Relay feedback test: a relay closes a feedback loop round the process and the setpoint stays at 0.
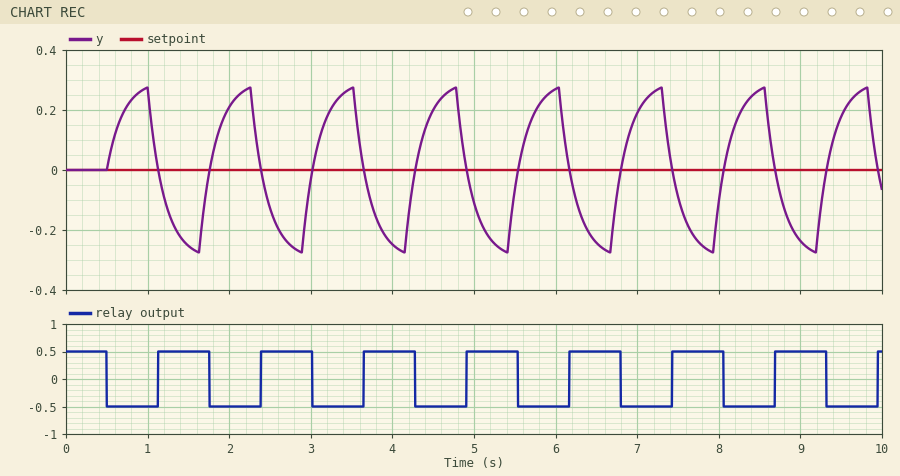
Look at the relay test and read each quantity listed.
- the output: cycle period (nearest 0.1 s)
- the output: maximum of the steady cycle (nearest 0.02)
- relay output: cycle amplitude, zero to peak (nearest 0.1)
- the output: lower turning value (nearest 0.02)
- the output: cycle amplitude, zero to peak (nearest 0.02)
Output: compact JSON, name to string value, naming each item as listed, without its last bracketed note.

{"the output: cycle period": "1.3 s", "the output: maximum of the steady cycle": "0.28", "relay output: cycle amplitude, zero to peak": "0.5", "the output: lower turning value": "-0.28", "the output: cycle amplitude, zero to peak": "0.28"}
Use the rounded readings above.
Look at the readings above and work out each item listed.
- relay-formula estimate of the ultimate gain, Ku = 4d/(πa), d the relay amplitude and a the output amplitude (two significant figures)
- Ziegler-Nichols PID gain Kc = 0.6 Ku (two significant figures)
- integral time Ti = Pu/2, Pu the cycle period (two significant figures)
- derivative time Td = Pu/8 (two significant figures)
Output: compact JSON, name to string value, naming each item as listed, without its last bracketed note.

{"relay-formula estimate of the ultimate gain, Ku = 4d/(πa), d the relay amplitude and a the output amplitude": "2.3", "Ziegler-Nichols PID gain Kc = 0.6 Ku": "1.4", "integral time Ti = Pu/2, Pu the cycle period": "0.65 s", "derivative time Td = Pu/8": "0.16 s"}
